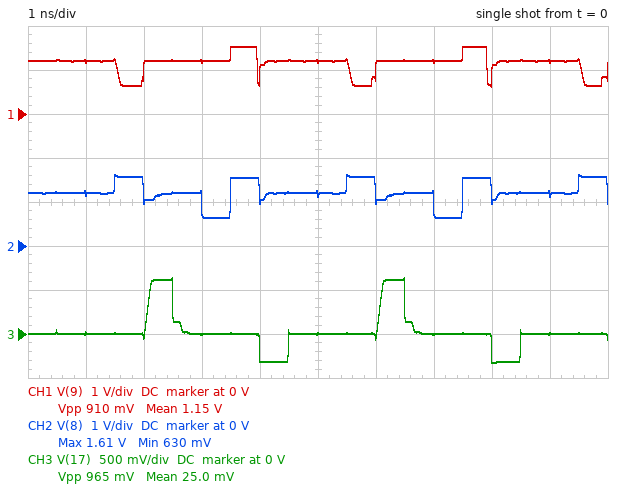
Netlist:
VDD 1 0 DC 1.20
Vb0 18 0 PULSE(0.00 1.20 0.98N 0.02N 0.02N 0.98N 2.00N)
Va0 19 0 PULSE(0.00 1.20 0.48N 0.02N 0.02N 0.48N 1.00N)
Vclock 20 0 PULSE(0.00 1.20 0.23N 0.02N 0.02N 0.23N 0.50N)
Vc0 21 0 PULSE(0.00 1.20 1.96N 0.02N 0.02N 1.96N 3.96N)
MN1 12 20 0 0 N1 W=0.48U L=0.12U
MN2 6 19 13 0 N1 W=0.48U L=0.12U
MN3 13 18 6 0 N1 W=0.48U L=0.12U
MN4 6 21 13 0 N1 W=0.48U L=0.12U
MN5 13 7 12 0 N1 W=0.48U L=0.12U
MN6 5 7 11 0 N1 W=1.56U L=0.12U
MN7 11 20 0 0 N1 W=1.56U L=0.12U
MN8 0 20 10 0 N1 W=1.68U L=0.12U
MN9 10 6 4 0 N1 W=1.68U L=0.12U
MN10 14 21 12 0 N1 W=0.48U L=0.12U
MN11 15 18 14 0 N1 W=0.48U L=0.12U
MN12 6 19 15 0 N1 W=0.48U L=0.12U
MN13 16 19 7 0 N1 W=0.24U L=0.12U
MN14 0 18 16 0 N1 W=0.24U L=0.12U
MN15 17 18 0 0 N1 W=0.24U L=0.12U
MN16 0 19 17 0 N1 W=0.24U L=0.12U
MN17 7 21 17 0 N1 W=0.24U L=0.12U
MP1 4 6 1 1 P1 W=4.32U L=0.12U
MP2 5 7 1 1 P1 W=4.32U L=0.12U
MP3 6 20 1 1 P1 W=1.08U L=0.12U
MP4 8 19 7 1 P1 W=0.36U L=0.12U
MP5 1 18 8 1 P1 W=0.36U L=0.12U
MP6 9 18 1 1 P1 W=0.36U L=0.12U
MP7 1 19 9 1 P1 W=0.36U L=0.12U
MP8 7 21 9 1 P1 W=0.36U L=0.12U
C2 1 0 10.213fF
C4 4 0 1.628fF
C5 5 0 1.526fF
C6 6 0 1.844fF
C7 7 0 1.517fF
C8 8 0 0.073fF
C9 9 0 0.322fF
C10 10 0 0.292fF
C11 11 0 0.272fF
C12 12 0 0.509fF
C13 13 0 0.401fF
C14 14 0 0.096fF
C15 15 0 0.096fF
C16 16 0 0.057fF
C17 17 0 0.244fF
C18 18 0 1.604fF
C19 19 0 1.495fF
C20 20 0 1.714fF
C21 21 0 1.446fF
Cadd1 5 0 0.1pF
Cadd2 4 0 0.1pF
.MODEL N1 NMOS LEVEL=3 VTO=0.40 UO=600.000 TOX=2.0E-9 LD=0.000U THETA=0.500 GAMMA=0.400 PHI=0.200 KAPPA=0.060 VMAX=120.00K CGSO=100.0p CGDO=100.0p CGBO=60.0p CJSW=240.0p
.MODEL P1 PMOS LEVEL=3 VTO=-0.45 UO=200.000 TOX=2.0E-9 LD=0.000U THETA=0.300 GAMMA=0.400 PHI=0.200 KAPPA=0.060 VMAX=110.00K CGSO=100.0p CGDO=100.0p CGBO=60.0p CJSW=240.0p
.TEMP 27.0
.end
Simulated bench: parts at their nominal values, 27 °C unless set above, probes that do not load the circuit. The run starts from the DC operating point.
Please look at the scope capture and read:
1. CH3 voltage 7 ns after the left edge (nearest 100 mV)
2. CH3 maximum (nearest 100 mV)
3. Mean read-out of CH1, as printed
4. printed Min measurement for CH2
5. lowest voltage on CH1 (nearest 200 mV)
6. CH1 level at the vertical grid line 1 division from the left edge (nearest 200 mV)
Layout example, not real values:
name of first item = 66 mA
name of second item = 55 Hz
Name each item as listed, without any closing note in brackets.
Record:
CH3 voltage 7 ns after the left edge = 0 V
CH3 maximum = 600 mV
Mean read-out of CH1, as printed = 1.15 V
printed Min measurement for CH2 = 630 mV
lowest voltage on CH1 = 600 mV
CH1 level at the vertical grid line 1 division from the left edge = 1.2 V
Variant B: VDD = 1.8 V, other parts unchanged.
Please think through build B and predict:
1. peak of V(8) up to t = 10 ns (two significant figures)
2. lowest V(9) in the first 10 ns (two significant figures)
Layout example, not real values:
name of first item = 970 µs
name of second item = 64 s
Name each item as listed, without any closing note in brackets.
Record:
peak of V(8) up to t = 10 ns = 1.9 V
lowest V(9) in the first 10 ns = 900 mV
